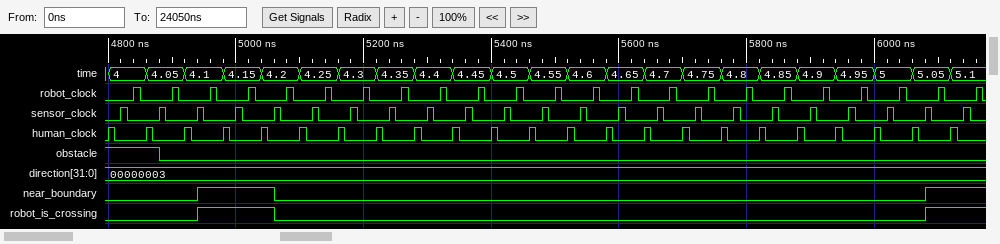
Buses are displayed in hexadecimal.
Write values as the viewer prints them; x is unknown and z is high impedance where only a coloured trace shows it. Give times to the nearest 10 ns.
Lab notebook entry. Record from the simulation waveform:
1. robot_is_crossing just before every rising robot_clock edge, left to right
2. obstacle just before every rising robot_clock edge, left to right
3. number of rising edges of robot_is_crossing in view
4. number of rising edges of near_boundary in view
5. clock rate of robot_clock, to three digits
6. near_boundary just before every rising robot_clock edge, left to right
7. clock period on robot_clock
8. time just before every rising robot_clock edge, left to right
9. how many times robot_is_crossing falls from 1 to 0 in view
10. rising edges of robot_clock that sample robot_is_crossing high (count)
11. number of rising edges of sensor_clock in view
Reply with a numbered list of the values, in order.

1. 0 0 1 1 0 0 0 0 0 0 0 0 0 0 0 0 0 0 0 0 0 1 1
2. 1 0 0 0 0 0 0 0 0 0 0 0 0 0 0 0 0 0 0 0 0 0 0
3. 2
4. 2
5. 16.7 MHz
6. 0 0 1 1 0 0 0 0 0 0 0 0 0 0 0 0 0 0 0 0 0 1 1
7. 60 ns
8. 4, 4.05, 4.1, 4.15, 4.2, 4.25, 4.3, 4.35, 4.4, 4.45, 4.5, 4.55, 4.6, 4.65, 4.7, 4.75, 4.8, 4.85, 4.9, 4.95, 5, 5.05, 5.1
9. 1
10. 4
11. 23
